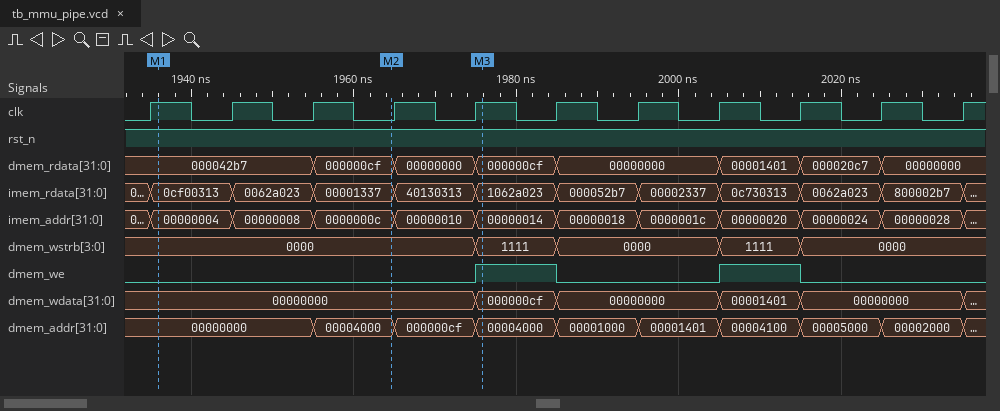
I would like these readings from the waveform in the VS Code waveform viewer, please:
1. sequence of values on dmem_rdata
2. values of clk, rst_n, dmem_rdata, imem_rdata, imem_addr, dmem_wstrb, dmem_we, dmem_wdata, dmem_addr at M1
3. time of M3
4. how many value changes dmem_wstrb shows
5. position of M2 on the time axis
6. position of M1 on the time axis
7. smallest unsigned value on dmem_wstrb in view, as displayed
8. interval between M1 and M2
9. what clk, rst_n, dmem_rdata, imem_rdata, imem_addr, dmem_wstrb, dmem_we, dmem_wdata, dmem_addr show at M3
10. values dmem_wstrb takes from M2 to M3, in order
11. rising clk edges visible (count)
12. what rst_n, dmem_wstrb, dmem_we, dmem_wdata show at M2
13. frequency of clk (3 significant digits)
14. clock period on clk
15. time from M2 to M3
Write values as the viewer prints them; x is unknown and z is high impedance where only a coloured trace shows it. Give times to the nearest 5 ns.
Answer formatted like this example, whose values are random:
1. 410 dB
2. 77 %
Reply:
1. 000042b7, 000000cf, 00000000, 000000cf, 00000000, 00001401, 000020c7, 00000000
2. clk=1, rst_n=1, dmem_rdata=000042b7, imem_rdata=0cf00313, imem_addr=00000004, dmem_wstrb=0000, dmem_we=0, dmem_wdata=00000000, dmem_addr=00000000
3. 1975 ns
4. 4
5. 1965 ns
6. 1935 ns
7. 0000
8. 30 ns
9. clk=1, rst_n=1, dmem_rdata=000000cf, imem_rdata=1062a023, imem_addr=00000014, dmem_wstrb=1111, dmem_we=1, dmem_wdata=000000cf, dmem_addr=00004000
10. 0000, 1111
11. 11
12. rst_n=1, dmem_wstrb=0000, dmem_we=0, dmem_wdata=00000000
13. 100 MHz
14. 10 ns
15. 10 ns
